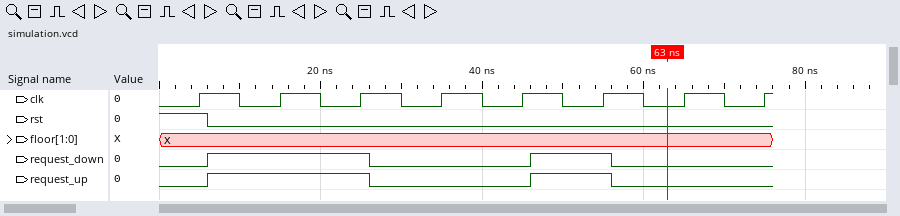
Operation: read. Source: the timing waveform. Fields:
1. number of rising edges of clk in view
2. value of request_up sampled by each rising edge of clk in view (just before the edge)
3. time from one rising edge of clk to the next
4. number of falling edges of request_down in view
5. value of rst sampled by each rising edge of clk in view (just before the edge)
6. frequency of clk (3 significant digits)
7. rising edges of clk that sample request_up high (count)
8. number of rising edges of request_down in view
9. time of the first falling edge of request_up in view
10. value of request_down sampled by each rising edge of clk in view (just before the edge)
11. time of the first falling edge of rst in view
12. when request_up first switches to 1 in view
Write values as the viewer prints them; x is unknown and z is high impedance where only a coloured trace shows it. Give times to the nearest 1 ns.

8
0 1 1 0 0 1 0 0
10 ns
2
1 0 0 0 0 0 0 0
100 MHz
3
2
26 ns
0 1 1 0 0 1 0 0
6 ns
6 ns
